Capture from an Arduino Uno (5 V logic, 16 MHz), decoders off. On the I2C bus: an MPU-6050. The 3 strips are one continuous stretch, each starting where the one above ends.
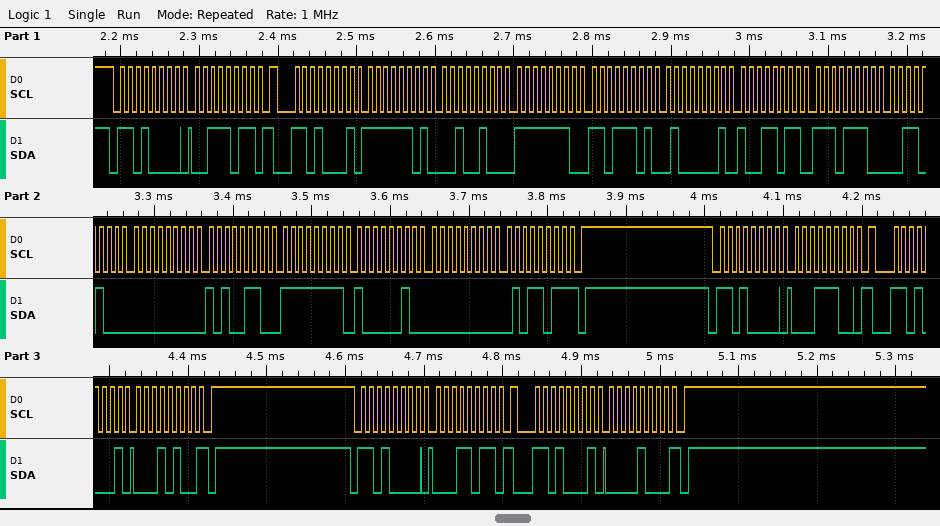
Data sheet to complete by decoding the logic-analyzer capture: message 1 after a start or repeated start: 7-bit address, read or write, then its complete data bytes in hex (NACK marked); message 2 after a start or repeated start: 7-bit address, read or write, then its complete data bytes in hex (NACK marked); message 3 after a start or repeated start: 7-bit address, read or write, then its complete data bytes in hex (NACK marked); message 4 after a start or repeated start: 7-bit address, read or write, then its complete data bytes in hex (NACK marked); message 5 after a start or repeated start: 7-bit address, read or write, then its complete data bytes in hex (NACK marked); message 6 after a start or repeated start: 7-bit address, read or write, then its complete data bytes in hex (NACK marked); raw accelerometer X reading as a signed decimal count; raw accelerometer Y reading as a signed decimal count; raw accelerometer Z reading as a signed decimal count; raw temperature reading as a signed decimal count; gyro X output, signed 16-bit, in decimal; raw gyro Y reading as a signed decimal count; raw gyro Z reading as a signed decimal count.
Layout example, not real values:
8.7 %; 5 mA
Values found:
0x68 write: 3B; 0x68 read: FD 24 FE DD 41 9B EE 34 00 A6 FF 82 00 5B NACK; 0x68 write: 1C; 0x68 read: 14 NACK; 0x68 write: 1B; 0x68 read: 08 NACK; -732; -291; 16795; -4556; 166; -126; 91
